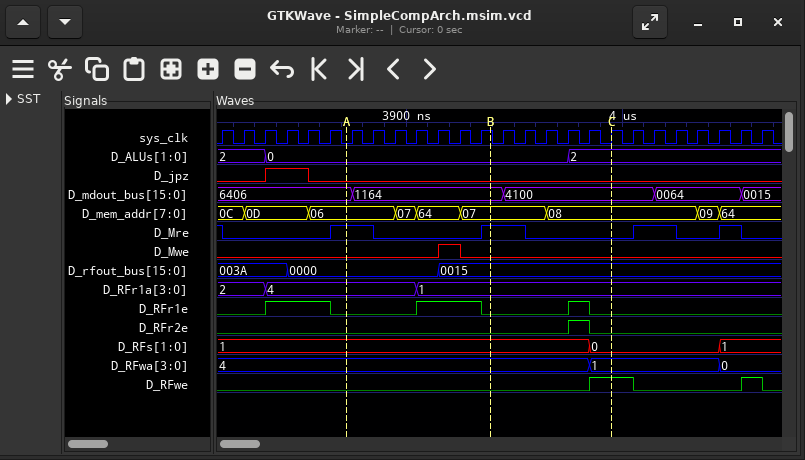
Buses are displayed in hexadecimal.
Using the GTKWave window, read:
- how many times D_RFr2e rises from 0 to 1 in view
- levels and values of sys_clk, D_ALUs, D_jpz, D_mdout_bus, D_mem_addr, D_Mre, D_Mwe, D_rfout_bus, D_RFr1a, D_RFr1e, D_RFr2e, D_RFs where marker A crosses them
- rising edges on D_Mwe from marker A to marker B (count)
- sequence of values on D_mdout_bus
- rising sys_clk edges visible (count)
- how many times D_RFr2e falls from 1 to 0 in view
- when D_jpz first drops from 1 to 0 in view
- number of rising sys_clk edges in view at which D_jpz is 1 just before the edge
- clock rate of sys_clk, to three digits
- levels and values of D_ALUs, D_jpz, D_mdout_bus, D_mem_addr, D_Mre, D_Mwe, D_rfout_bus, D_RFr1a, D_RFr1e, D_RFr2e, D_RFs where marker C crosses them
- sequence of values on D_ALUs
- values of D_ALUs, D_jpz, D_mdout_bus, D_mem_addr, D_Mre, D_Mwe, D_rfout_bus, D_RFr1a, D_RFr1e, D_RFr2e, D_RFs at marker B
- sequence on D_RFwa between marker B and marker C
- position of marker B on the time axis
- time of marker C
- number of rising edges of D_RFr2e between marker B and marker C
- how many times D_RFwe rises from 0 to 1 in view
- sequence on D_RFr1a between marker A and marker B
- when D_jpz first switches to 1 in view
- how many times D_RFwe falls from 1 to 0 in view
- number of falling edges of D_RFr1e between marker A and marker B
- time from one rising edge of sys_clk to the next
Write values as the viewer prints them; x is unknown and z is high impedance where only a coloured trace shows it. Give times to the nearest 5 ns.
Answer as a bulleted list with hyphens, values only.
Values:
- 1
- sys_clk=0, D_ALUs=0, D_jpz=0, D_mdout_bus=6406, D_mem_addr=06, D_Mre=1, D_Mwe=0, D_rfout_bus=0000, D_RFr1a=4, D_RFr1e=0, D_RFr2e=0, D_RFs=1
- 1
- 6406, 1164, 4100, 0064, 0015
- 26
- 1
- 3855 ns
- 2
- 100 MHz
- D_ALUs=2, D_jpz=0, D_mdout_bus=4100, D_mem_addr=08, D_Mre=0, D_Mwe=0, D_rfout_bus=0015, D_RFr1a=1, D_RFr1e=0, D_RFr2e=0, D_RFs=0
- 2, 0, 2
- D_ALUs=0, D_jpz=0, D_mdout_bus=1164, D_mem_addr=07, D_Mre=1, D_Mwe=0, D_rfout_bus=0015, D_RFr1a=1, D_RFr1e=0, D_RFr2e=0, D_RFs=1
- 4, 1
- 3940 ns
- 3995 ns
- 1
- 2
- 4, 1
- 3835 ns
- 2
- 1
- 10 ns
